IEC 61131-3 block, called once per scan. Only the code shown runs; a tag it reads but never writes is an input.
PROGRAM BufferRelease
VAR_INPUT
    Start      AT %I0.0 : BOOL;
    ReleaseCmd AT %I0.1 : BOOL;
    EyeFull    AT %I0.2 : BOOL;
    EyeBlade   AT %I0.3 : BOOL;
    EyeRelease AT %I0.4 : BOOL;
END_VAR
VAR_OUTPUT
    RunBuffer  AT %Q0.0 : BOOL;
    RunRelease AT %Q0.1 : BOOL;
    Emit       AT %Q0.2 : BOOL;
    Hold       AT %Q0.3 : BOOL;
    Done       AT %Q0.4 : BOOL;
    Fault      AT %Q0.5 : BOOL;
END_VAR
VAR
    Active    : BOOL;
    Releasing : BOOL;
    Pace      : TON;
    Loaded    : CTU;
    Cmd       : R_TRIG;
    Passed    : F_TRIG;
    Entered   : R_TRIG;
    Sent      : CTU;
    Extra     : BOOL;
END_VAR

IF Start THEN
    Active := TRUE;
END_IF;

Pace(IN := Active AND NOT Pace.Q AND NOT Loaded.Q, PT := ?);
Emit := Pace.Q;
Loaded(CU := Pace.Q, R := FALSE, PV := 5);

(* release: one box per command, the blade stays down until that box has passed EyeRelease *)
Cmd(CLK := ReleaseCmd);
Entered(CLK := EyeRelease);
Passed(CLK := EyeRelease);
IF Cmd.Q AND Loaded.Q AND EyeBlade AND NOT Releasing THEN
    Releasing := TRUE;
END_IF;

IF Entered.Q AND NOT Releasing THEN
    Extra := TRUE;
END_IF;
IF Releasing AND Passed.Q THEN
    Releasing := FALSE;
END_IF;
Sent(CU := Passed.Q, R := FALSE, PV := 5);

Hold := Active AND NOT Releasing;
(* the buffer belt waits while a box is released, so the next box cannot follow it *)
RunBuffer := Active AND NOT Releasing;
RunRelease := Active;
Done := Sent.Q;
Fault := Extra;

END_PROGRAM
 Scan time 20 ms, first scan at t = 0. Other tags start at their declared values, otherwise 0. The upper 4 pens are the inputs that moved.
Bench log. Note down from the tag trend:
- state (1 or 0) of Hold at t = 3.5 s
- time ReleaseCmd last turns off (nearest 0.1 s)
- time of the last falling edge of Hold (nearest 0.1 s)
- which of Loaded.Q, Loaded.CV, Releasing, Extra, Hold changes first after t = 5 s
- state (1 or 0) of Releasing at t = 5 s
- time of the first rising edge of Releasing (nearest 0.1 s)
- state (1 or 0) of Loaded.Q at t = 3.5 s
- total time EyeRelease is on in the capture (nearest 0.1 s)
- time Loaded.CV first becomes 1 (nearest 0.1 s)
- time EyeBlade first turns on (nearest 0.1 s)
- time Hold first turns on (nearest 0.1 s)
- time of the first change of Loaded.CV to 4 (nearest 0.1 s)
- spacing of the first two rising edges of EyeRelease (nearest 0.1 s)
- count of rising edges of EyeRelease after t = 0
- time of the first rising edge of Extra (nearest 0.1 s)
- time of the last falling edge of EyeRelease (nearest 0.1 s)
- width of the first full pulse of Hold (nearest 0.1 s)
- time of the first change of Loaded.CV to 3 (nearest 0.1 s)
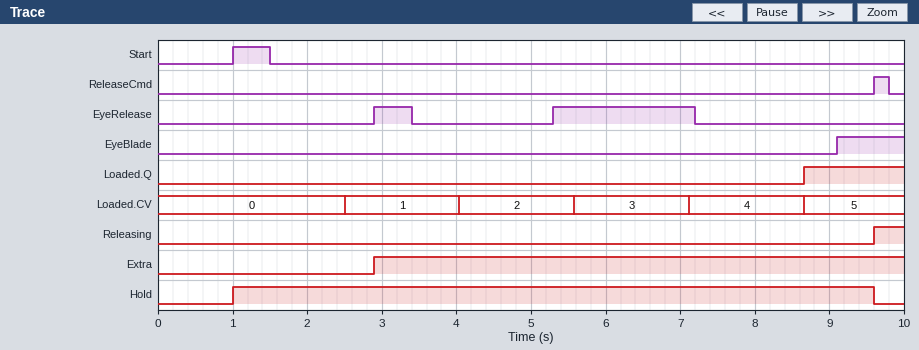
1
9.8 s
9.6 s
Loaded.CV
0
9.6 s
0
2.4 s
2.5 s
9.1 s
1.0 s
7.1 s
2.4 s
2
2.9 s
7.2 s
8.6 s
5.6 s
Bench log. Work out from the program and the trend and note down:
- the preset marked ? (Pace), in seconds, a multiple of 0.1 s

1.5 s
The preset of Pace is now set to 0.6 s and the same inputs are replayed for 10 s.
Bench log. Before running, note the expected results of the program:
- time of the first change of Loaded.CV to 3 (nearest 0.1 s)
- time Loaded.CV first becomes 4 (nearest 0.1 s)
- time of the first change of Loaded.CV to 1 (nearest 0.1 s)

2.9 s
3.5 s
1.6 s
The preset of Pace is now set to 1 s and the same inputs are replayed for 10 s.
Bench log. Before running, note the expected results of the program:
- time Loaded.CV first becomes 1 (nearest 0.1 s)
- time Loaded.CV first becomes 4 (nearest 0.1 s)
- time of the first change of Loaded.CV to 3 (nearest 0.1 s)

2.0 s
5.1 s
4.1 s
